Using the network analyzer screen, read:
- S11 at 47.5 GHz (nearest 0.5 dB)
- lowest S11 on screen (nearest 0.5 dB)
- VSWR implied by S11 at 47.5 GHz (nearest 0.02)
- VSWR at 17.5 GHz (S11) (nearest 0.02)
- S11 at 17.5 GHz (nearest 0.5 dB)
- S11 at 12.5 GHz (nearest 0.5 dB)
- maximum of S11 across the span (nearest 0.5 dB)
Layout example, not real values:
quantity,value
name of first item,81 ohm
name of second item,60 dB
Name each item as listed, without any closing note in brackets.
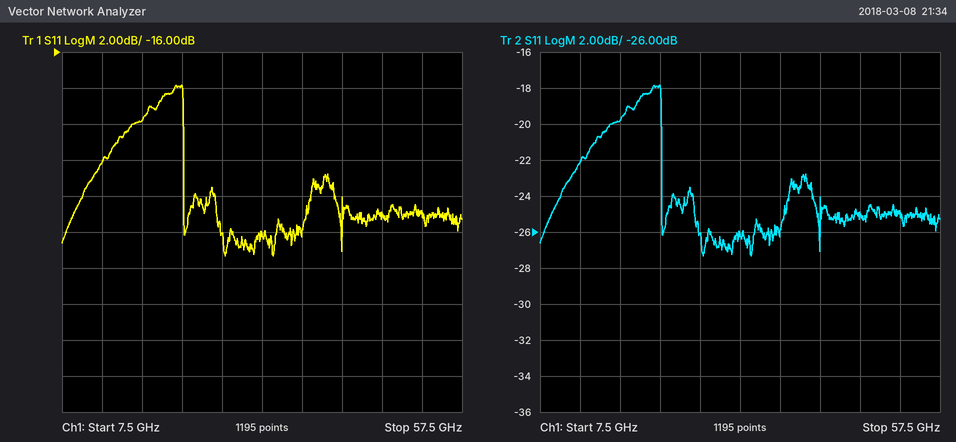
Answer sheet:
quantity,value
S11 at 47.5 GHz,-25.0 dB
lowest S11 on screen,-27.5 dB
VSWR implied by S11 at 47.5 GHz,1.12
VSWR at 17.5 GHz (S11),1.22
S11 at 17.5 GHz,-20.0 dB
S11 at 12.5 GHz,-22.0 dB
maximum of S11 across the span,-18.0 dB
